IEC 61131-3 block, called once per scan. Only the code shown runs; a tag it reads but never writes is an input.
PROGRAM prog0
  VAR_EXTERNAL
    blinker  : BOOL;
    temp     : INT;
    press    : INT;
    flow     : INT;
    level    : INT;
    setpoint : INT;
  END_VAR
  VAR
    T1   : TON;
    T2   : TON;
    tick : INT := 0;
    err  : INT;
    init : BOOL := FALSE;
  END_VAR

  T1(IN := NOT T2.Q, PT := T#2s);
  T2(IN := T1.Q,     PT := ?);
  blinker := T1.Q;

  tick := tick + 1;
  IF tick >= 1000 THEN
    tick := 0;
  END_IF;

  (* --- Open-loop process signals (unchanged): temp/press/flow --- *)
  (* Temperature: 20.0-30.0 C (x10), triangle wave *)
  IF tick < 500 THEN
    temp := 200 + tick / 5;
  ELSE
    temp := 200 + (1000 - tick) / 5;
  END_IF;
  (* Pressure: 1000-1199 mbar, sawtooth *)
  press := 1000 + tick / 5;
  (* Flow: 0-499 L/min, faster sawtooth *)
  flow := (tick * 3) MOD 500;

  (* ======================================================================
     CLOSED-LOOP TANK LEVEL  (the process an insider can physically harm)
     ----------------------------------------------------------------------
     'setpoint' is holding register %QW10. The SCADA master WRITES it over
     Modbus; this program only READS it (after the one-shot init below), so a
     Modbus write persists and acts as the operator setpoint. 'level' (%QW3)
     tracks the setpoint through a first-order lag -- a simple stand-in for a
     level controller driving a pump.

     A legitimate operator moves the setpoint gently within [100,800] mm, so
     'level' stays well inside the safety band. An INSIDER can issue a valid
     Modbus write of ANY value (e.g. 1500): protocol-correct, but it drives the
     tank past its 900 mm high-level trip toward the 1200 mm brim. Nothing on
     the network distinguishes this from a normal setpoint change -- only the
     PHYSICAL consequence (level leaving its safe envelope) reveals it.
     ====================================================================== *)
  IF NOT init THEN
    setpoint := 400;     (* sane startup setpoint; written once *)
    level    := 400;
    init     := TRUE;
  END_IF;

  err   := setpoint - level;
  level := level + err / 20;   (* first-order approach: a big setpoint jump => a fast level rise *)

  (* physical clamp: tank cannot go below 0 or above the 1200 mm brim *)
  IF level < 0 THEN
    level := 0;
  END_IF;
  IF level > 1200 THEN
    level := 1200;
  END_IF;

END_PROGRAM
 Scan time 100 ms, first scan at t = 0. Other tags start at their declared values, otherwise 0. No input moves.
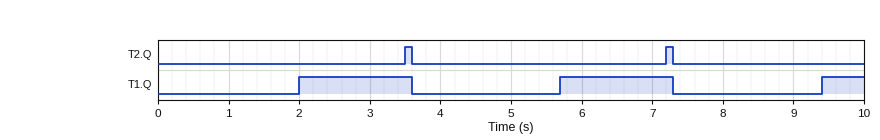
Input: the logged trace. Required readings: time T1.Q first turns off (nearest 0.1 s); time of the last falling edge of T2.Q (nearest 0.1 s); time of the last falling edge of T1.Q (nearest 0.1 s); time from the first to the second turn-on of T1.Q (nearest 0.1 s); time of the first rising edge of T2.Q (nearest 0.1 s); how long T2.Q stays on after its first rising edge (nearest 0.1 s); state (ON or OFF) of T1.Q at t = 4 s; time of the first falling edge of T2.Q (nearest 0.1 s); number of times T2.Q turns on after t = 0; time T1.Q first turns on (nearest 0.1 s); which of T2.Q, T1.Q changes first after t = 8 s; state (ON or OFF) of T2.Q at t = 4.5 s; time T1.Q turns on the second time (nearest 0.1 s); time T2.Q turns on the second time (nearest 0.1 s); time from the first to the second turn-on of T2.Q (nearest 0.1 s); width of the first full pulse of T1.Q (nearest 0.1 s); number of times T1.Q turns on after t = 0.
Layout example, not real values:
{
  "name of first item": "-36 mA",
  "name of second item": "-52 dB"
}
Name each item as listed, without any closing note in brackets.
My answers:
{
  "time T1.Q first turns off": "3.6 s",
  "time of the last falling edge of T2.Q": "7.3 s",
  "time of the last falling edge of T1.Q": "7.3 s",
  "time from the first to the second turn-on of T1.Q": "3.7 s",
  "time of the first rising edge of T2.Q": "3.5 s",
  "how long T2.Q stays on after its first rising edge": "0.1 s",
  "state (ON or OFF) of T1.Q at t = 4 s": "OFF",
  "time of the first falling edge of T2.Q": "3.6 s",
  "number of times T2.Q turns on after t = 0": "2",
  "time T1.Q first turns on": "2.0 s",
  "which of T2.Q, T1.Q changes first after t = 8 s": "T1.Q",
  "state (ON or OFF) of T2.Q at t = 4.5 s": "OFF",
  "time T1.Q turns on the second time": "5.7 s",
  "time T2.Q turns on the second time": "7.2 s",
  "time from the first to the second turn-on of T2.Q": "3.7 s",
  "width of the first full pulse of T1.Q": "1.6 s",
  "number of times T1.Q turns on after t = 0": "3"
}
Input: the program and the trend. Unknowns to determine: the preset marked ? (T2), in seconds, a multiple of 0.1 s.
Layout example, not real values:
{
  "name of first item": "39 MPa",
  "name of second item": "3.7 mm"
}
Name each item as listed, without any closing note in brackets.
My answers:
{
  "the preset marked ? (T2), in seconds, a multiple of 0.1 s": "1.5 s"
}
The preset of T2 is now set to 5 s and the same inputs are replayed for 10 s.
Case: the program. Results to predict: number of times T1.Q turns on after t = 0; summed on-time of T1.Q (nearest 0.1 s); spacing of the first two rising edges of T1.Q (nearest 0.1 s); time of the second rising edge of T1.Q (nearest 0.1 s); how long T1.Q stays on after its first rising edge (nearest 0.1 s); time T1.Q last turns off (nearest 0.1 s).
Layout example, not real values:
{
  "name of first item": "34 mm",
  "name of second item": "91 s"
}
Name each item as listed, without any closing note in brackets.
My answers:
{
  "number of times T1.Q turns on after t = 0": "2",
  "summed on-time of T1.Q": "5.9 s",
  "spacing of the first two rising edges of T1.Q": "7.2 s",
  "time of the second rising edge of T1.Q": "9.2 s",
  "how long T1.Q stays on after its first rising edge": "5.1 s",
  "time T1.Q last turns off": "7.1 s"
}
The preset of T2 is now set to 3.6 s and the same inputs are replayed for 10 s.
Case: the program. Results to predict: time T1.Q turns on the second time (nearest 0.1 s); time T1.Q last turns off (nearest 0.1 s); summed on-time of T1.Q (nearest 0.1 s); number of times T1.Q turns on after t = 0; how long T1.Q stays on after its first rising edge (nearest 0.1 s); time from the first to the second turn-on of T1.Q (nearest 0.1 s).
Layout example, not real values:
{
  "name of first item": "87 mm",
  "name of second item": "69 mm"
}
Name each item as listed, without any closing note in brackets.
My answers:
{
  "time T1.Q turns on the second time": "7.8 s",
  "time T1.Q last turns off": "5.7 s",
  "summed on-time of T1.Q": "5.9 s",
  "number of times T1.Q turns on after t = 0": "2",
  "how long T1.Q stays on after its first rising edge": "3.7 s",
  "time from the first to the second turn-on of T1.Q": "5.8 s"
}
